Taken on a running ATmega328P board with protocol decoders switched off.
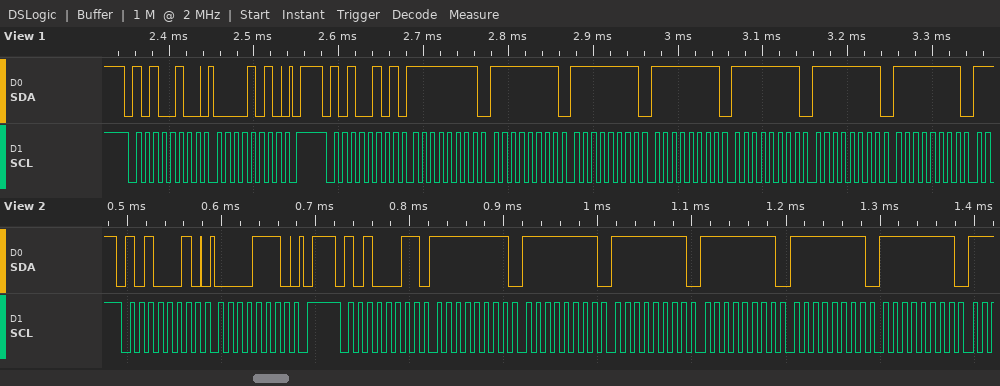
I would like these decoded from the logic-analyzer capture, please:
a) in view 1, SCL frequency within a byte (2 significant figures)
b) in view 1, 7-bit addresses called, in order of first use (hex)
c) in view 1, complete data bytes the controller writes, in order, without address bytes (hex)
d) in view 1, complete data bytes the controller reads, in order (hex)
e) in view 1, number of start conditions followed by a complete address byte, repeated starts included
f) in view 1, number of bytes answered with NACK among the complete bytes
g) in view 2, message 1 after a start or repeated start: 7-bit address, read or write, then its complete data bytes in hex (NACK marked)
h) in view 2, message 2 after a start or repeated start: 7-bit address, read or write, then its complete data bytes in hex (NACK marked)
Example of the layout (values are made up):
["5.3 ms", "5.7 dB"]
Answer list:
["100 kHz", "0x52", "0A", "FF FF FF FF FF FF FF", "2", "0", "0x51 write: 0E", "0x51 read: FF FF FF FF FF FF"]
